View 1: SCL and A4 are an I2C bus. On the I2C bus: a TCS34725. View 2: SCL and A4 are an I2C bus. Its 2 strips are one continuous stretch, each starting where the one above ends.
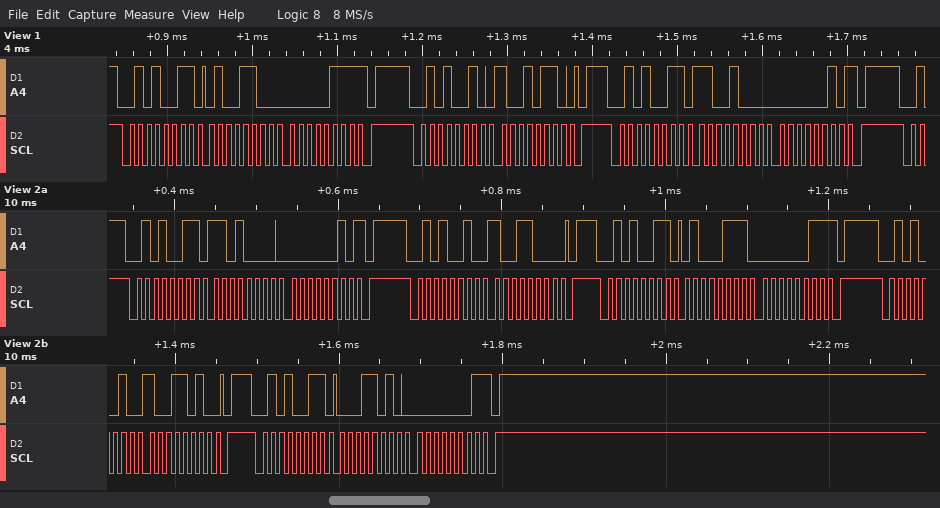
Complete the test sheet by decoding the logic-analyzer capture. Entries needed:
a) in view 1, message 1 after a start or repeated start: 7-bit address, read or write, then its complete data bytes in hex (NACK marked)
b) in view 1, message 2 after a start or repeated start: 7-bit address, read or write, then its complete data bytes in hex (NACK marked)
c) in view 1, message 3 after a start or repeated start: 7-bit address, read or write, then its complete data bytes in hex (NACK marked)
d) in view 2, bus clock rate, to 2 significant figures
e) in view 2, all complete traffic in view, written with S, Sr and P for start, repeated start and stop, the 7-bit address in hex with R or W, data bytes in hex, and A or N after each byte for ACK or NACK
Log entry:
0x29 read: 4C 07 NACK
0x29 write: 96
0x29 read: C8 02 NACK
100 kHz
S 29R A D0 A 02 N P S 29W A 98 A P S 29R A 47 A 03 N P S 29W A 9A A P S 29R A 1A A 01 N P
